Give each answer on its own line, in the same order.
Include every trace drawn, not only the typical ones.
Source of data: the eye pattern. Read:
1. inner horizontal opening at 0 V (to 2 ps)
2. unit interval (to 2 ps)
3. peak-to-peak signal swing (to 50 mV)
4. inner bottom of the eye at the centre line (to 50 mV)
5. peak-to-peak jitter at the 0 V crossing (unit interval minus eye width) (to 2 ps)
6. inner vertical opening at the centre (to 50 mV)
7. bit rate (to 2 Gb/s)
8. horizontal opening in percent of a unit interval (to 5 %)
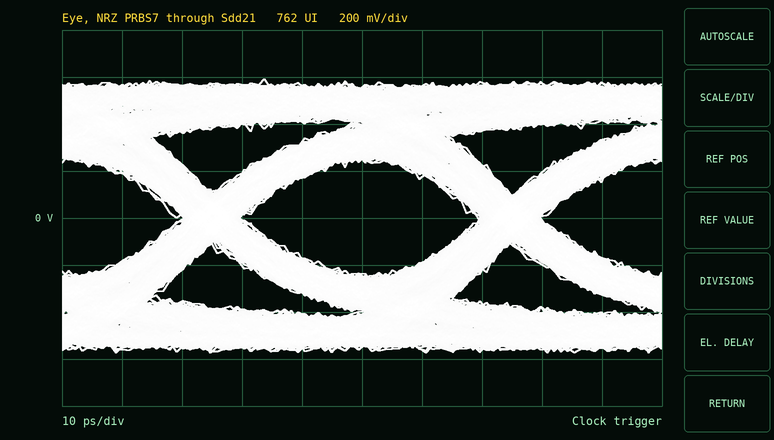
40 ps
50 ps
1.15 V
-250 mV
10 ps
500 mV
20 Gb/s
80 %
